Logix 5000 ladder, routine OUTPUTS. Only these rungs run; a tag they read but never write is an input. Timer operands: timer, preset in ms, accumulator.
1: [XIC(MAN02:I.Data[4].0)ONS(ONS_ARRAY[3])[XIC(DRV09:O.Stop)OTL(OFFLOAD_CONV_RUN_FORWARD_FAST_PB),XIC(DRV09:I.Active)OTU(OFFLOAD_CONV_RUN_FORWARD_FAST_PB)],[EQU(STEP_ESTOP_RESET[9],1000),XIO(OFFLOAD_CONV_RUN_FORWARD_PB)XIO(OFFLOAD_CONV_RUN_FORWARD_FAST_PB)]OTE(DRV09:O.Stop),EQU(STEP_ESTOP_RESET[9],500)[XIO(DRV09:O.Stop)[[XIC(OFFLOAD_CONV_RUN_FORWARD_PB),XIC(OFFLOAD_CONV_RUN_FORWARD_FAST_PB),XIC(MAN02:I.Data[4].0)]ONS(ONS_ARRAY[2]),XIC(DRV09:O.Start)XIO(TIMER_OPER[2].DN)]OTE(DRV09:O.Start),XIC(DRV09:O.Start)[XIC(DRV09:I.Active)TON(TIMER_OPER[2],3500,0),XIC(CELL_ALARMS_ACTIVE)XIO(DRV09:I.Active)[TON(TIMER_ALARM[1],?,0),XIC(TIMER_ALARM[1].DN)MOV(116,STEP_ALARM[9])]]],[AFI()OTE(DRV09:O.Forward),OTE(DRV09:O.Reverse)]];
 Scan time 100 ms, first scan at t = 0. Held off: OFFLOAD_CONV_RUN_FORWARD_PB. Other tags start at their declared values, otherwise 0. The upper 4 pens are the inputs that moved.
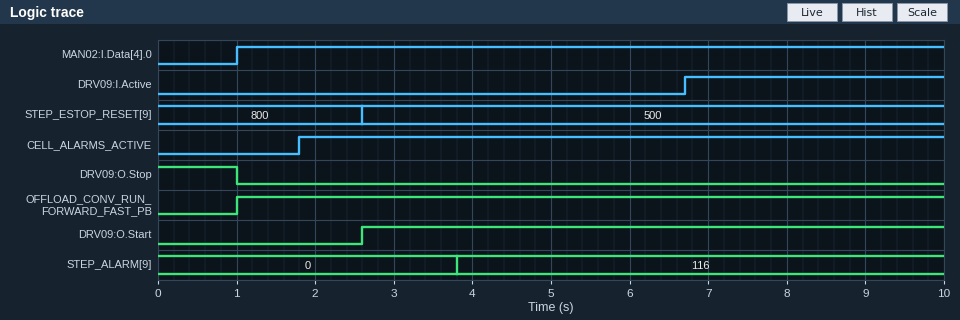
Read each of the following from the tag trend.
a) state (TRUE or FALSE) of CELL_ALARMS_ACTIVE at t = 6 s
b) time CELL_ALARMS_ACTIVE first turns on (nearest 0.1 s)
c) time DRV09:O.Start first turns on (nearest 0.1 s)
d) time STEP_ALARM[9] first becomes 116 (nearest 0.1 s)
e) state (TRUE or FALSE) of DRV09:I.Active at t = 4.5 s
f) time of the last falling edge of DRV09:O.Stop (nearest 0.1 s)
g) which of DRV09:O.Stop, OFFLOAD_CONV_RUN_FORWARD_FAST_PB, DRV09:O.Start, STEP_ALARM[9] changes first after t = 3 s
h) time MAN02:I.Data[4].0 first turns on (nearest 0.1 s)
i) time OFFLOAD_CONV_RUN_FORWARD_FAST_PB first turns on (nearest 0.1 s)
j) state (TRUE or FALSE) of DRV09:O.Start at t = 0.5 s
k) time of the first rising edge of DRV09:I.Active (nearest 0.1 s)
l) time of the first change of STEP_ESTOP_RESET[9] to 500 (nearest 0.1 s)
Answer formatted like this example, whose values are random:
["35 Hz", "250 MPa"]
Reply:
["TRUE", "1.8 s", "2.6 s", "3.8 s", "FALSE", "1.0 s", "STEP_ALARM[9]", "1.0 s", "1.0 s", "FALSE", "6.7 s", "2.6 s"]
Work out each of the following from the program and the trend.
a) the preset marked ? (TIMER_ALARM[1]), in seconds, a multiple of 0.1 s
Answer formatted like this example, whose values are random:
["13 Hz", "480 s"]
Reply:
["1.2 s"]
